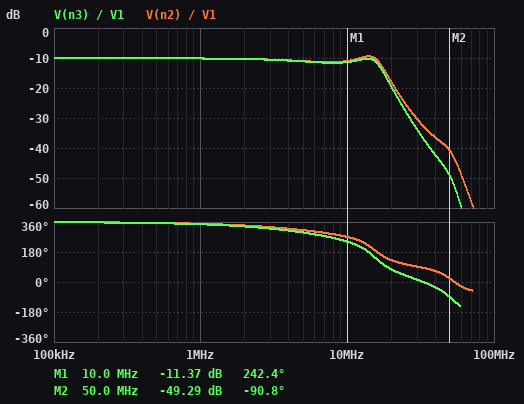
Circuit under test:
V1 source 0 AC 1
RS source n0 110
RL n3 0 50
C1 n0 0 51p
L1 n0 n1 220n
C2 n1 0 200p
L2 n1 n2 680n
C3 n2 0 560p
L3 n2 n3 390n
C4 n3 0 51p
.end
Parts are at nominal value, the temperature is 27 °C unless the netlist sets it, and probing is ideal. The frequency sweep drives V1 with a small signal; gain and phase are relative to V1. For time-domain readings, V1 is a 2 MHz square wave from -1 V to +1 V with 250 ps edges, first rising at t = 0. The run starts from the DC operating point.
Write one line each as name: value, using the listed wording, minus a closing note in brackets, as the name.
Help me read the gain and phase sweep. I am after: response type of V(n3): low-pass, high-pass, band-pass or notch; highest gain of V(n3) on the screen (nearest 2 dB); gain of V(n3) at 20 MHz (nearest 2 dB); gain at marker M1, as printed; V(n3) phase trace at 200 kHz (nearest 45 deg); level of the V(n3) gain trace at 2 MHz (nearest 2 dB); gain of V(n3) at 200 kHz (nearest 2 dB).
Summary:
response type of V(n3): low-pass, high-pass, band-pass or notch: low-pass
highest gain of V(n3) on the screen: -10 dB
gain of V(n3) at 20 MHz: -20 dB
gain at marker M1, as printed: -11.37 dB
V(n3) phase trace at 200 kHz: 360 deg
level of the V(n3) gain trace at 2 MHz: -10 dB
gain of V(n3) at 200 kHz: -10 dB
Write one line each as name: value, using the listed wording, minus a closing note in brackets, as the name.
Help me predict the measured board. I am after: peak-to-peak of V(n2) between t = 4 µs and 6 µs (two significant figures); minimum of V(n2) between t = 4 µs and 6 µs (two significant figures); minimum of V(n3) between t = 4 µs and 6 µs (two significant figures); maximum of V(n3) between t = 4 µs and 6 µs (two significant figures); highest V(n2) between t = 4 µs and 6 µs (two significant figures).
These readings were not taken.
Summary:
peak-to-peak of V(n2) between t = 4 µs and 6 µs: 700 mV
minimum of V(n2) between t = 4 µs and 6 µs: -350 mV
minimum of V(n3) between t = 4 µs and 6 µs: -340 mV
maximum of V(n3) between t = 4 µs and 6 µs: 340 mV
highest V(n2) between t = 4 µs and 6 µs: 350 mV
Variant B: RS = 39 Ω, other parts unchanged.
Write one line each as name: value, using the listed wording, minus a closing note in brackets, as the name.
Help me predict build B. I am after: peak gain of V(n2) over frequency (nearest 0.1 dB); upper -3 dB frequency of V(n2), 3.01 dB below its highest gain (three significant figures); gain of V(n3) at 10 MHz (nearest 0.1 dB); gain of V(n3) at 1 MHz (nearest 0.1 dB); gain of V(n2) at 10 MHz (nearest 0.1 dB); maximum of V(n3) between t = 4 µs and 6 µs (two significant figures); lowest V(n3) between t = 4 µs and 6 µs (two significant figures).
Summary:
peak gain of V(n2) over frequency: -4.9 dB
upper -3 dB frequency of V(n2), 3.01 dB below its highest gain: 14.8 MHz
gain of V(n3) at 10 MHz: -5.8 dB
gain of V(n3) at 1 MHz: -5.0 dB
gain of V(n2) at 10 MHz: -5.5 dB
maximum of V(n3) between t = 4 µs and 6 µs: 640 mV
lowest V(n3) between t = 4 µs and 6 µs: -640 mV
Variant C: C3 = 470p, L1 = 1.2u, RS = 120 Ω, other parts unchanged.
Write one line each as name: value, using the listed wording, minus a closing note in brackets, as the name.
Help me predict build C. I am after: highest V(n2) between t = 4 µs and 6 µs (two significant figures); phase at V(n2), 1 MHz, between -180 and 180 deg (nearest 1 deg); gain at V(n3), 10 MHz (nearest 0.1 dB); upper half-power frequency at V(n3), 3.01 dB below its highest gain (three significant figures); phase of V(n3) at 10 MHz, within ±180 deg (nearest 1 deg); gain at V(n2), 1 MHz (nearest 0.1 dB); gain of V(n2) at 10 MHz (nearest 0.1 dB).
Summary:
highest V(n2) between t = 4 µs and 6 µs: 360 mV
phase at V(n2), 1 MHz, between -180 and 180 deg: -12 deg
gain at V(n3), 10 MHz: -11.9 dB
upper half-power frequency at V(n3), 3.01 dB below its highest gain: 20.2 MHz
phase of V(n3) at 10 MHz, within ±180 deg: -138 deg
gain at V(n2), 1 MHz: -10.7 dB
gain of V(n2) at 10 MHz: -11.5 dB
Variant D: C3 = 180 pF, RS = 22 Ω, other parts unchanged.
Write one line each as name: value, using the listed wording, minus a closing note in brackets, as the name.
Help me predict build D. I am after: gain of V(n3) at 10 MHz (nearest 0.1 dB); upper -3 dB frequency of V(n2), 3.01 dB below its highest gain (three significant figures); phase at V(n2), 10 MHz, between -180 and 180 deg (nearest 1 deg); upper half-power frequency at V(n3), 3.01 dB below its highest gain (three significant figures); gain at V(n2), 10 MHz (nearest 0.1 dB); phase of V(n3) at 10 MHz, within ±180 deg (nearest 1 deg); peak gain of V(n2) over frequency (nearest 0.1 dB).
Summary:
gain of V(n3) at 10 MHz: -3.6 dB
upper -3 dB frequency of V(n2), 3.01 dB below its highest gain: 31.1 MHz
phase at V(n2), 10 MHz, between -180 and 180 deg: -61 deg
upper half-power frequency at V(n3), 3.01 dB below its highest gain: 29.7 MHz
gain at V(n2), 10 MHz: -3.2 dB
phase of V(n3) at 10 MHz, within ±180 deg: -89 deg
peak gain of V(n2) over frequency: -1.2 dB
